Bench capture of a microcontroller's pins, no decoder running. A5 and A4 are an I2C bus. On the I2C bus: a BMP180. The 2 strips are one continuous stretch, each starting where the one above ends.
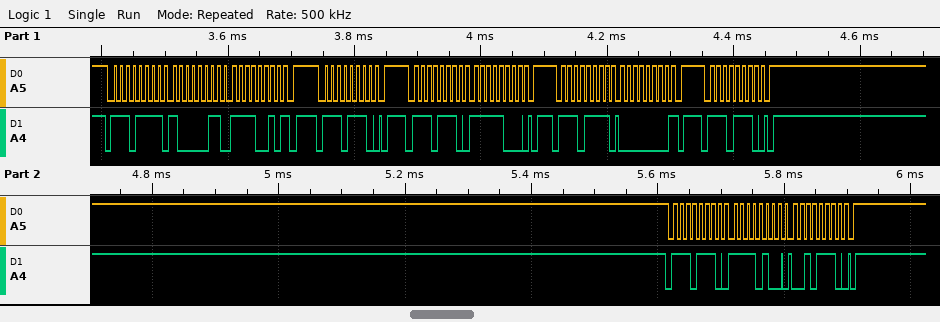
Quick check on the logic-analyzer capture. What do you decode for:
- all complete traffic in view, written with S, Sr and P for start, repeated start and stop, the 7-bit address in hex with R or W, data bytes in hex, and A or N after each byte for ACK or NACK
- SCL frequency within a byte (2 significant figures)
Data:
S 77R A 83 A F2 N P S 77W A P S 77W A F8 A P S 77R A 00 N P S 77W A P S 77W A F4 A 2E A P
100 kHz
